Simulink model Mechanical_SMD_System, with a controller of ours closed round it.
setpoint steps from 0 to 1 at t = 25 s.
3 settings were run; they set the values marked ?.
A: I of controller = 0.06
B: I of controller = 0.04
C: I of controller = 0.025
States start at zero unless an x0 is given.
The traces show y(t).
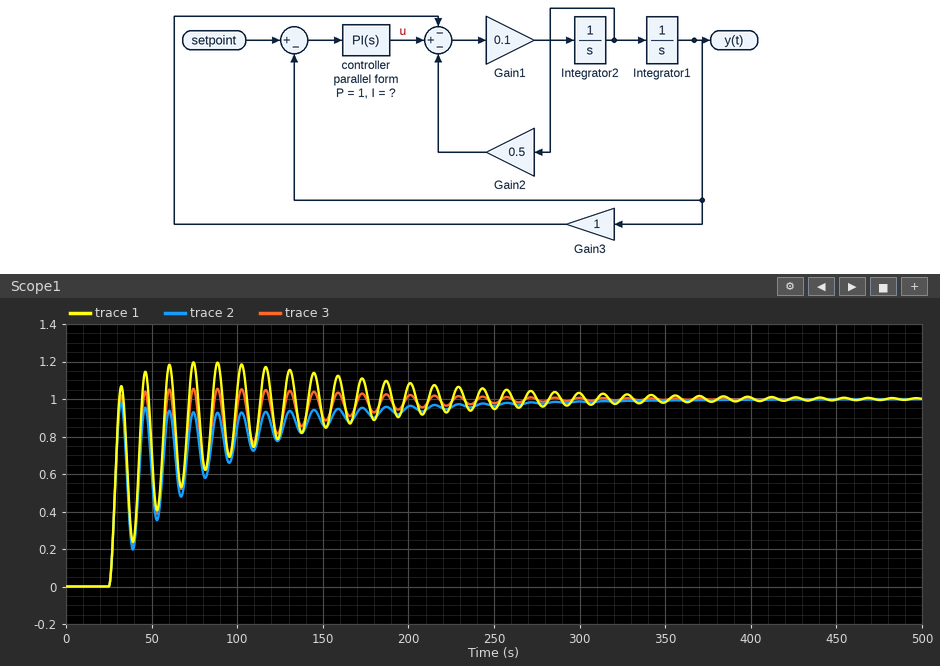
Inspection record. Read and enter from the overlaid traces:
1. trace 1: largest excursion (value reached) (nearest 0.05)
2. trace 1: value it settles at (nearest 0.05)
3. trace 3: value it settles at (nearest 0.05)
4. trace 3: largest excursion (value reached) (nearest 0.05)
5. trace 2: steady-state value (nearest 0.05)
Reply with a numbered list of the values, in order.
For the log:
1. 1.20
2. 1.00
3. 1.00
4. 1.05
5. 1.00
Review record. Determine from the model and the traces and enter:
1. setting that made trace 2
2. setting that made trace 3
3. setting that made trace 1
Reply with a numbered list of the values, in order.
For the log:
1. C
2. B
3. A
